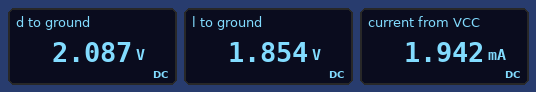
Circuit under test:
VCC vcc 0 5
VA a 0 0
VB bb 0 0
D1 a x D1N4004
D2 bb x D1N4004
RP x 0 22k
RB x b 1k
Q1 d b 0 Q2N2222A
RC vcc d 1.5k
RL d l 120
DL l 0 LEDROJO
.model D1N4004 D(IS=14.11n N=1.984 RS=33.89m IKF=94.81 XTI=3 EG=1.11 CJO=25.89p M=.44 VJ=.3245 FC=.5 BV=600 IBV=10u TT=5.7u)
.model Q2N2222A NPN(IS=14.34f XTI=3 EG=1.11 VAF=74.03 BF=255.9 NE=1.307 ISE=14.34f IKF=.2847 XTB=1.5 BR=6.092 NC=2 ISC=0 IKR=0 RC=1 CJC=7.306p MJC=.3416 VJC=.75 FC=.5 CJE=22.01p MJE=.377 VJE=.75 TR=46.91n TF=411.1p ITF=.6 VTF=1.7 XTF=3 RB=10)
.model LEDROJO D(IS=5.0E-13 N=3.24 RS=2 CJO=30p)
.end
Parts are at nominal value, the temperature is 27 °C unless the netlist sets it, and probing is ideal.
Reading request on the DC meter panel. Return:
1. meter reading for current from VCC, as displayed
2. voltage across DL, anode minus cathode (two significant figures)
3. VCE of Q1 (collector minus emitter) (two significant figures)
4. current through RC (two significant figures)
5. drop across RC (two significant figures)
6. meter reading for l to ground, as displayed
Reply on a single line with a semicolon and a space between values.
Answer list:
1.942 mA; 1.9 V; 2.1 V; 1.9 mA; 2.9 V; 1.854 V
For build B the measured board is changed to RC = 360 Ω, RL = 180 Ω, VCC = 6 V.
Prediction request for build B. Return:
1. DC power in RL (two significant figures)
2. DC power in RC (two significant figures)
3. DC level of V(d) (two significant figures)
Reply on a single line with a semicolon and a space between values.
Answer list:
10 mW; 20 mW; 3.3 V
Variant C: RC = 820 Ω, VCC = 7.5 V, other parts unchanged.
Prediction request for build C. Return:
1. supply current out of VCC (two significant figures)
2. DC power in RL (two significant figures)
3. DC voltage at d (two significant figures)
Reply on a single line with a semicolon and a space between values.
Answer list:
5.9 mA; 4.2 mW; 2.7 V
